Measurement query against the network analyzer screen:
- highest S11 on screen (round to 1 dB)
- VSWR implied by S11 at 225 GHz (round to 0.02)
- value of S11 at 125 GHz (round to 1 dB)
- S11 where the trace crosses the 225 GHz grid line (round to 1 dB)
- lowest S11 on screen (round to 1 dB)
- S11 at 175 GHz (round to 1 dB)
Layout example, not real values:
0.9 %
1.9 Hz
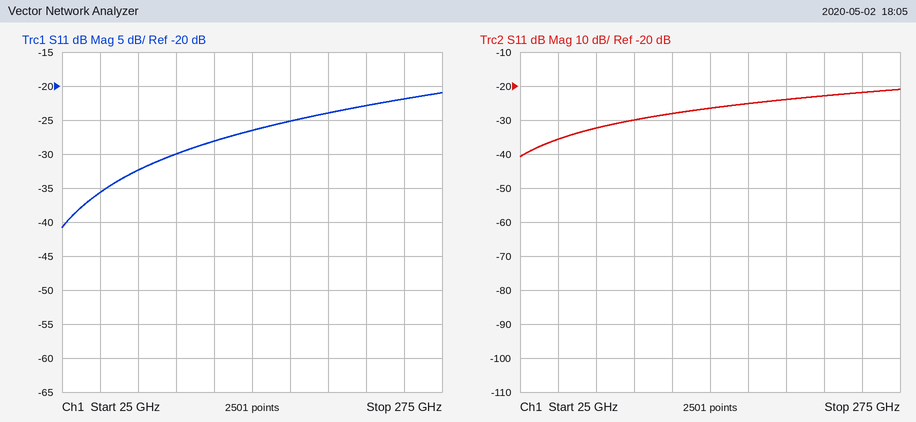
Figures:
-21 dB
1.16
-28 dB
-23 dB
-41 dB
-25 dB
